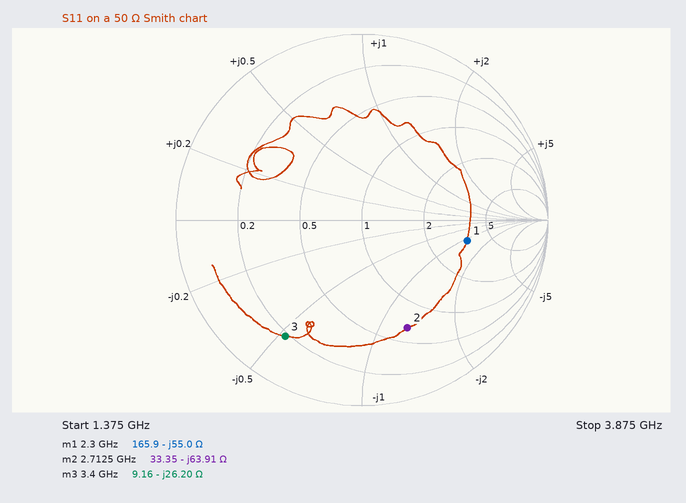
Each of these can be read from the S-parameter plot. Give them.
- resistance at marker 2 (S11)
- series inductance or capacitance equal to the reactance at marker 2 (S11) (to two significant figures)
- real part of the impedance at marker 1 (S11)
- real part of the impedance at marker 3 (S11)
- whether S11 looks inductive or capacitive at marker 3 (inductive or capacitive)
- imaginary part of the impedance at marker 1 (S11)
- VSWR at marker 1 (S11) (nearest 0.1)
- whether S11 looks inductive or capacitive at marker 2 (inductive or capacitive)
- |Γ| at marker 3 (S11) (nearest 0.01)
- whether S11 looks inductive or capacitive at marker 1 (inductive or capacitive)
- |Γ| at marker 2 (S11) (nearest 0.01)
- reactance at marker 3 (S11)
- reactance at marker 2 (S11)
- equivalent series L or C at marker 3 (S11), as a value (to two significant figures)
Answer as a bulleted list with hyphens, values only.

- 33.35 Ω
- 920 fF
- 165.9 Ω
- 9.16 Ω
- capacitive
- -55.0 Ω
- 3.7
- capacitive
- 0.75
- capacitive
- 0.63
- -26.20 Ω
- -63.91 Ω
- 1.8 pF
